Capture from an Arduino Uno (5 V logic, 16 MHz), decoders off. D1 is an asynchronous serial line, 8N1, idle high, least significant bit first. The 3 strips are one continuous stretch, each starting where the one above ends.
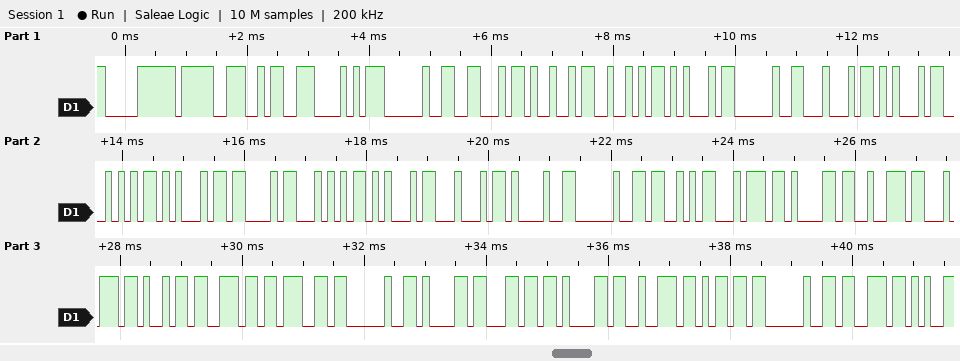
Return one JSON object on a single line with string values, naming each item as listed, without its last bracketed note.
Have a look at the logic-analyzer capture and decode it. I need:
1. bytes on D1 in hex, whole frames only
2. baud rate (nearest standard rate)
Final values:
{"bytes on D1 in hex, whole frames only": "F0 9F 9A A8 20 46 49 52 45 20 44 45 54 45 43 54 45 44 21 20 53 74 61 72 74 69 6E 67 20 61 6C 61 72 6D 20 73", "baud rate": "9600 baud"}
